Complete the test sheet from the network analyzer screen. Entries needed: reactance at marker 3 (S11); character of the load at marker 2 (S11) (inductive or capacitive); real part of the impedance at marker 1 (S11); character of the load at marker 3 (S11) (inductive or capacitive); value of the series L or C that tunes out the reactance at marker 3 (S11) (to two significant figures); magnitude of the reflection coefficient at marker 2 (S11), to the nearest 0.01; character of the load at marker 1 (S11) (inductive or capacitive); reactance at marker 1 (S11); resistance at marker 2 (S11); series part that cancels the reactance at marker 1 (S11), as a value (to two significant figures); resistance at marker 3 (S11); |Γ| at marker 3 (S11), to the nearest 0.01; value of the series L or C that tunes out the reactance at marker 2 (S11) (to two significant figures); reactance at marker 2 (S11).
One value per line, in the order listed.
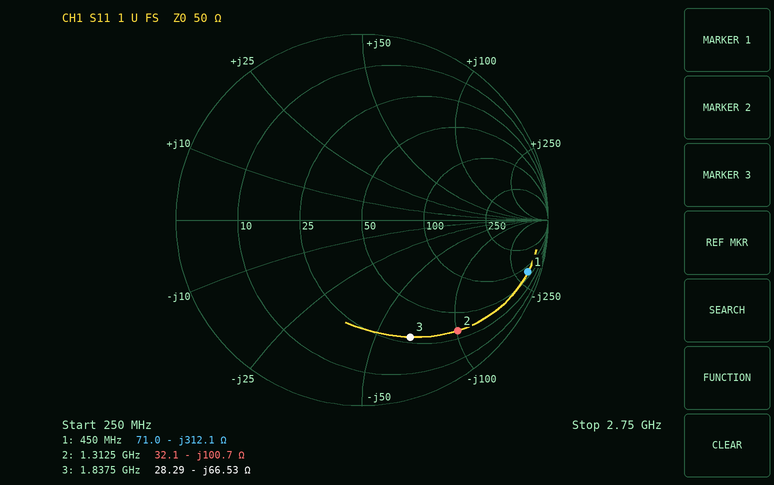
-66.53 Ω
capacitive
71.0 Ω
capacitive
5.8 nH
0.79
capacitive
-312.1 Ω
32.1 Ω
110 nH
28.29 Ω
0.68
12 nH
-100.7 Ω
